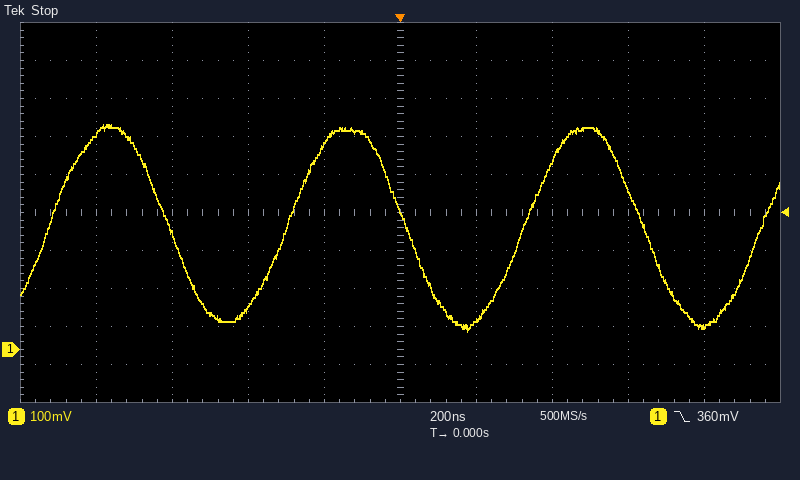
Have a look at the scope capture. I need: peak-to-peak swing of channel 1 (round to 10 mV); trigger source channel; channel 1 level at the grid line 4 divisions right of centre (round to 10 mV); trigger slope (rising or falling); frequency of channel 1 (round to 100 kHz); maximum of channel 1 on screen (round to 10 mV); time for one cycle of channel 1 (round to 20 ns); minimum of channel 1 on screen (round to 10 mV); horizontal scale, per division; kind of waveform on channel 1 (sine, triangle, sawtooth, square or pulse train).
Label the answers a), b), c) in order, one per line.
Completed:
a) 540 mV
b) channel 1
c) 60 mV
d) falling
e) 1.6 MHz
f) 590 mV
g) 620 ns
h) 50 mV
i) 200 ns
j) sine
